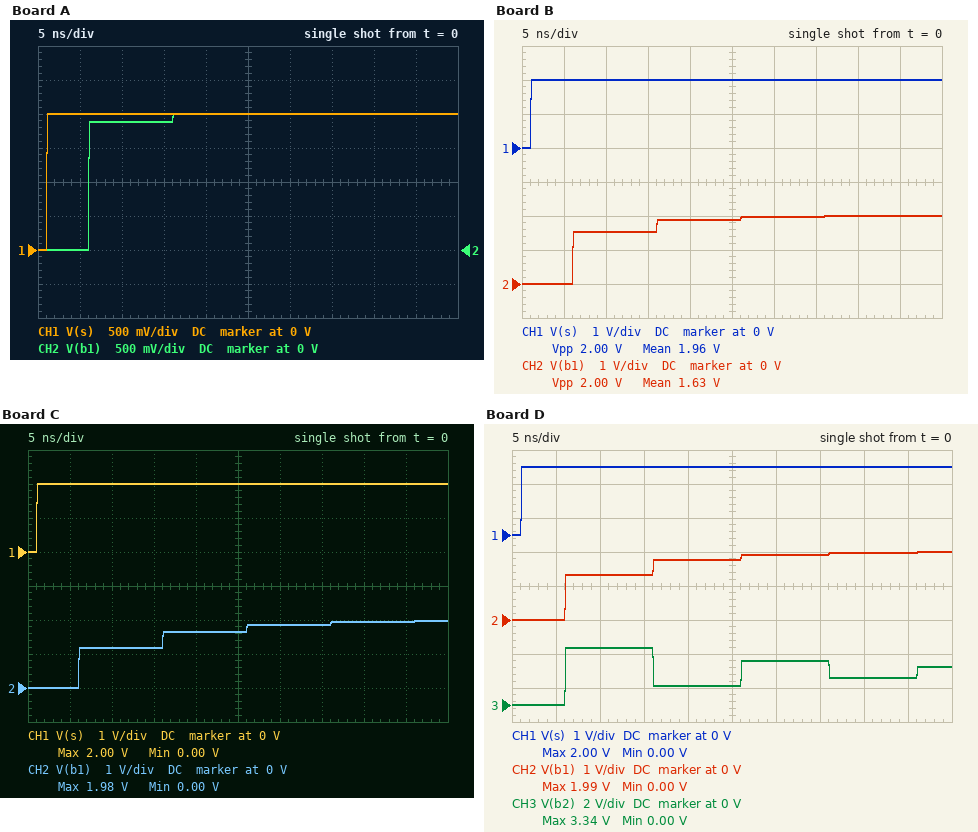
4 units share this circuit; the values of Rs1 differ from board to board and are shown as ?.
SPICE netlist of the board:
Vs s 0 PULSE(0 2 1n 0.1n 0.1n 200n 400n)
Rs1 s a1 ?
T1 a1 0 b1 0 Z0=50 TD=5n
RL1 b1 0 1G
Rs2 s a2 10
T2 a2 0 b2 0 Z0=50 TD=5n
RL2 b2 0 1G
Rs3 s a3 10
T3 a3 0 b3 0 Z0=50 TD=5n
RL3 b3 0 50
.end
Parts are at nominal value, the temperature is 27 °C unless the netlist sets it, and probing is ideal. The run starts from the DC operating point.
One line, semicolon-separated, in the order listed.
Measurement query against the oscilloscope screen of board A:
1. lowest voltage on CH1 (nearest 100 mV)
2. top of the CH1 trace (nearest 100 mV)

0 V; 2.0 V
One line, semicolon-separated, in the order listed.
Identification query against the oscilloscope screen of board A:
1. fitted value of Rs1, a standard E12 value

56 Ω
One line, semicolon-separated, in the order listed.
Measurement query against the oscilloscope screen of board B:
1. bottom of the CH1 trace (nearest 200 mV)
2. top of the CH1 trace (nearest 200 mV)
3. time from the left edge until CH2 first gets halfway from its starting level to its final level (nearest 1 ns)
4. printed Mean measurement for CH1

0 V; 2.0 V; 6 ns; 1.96 V
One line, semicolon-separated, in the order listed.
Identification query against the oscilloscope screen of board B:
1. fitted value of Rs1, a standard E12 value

82 Ω
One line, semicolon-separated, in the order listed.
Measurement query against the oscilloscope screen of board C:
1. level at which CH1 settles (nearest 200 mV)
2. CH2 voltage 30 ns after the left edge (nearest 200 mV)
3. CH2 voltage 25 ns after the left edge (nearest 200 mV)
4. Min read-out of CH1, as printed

2.0 V; 1.8 V; 1.6 V; 0.00 V
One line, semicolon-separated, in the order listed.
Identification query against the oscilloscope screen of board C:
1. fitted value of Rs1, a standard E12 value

120 Ω
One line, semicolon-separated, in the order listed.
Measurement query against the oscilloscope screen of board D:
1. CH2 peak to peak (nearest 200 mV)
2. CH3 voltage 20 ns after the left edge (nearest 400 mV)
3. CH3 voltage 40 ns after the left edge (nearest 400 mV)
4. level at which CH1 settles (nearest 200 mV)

2.0 V; 1.2 V; 1.6 V; 2.0 V
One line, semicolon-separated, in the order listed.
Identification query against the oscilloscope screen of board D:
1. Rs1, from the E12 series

100 Ω
